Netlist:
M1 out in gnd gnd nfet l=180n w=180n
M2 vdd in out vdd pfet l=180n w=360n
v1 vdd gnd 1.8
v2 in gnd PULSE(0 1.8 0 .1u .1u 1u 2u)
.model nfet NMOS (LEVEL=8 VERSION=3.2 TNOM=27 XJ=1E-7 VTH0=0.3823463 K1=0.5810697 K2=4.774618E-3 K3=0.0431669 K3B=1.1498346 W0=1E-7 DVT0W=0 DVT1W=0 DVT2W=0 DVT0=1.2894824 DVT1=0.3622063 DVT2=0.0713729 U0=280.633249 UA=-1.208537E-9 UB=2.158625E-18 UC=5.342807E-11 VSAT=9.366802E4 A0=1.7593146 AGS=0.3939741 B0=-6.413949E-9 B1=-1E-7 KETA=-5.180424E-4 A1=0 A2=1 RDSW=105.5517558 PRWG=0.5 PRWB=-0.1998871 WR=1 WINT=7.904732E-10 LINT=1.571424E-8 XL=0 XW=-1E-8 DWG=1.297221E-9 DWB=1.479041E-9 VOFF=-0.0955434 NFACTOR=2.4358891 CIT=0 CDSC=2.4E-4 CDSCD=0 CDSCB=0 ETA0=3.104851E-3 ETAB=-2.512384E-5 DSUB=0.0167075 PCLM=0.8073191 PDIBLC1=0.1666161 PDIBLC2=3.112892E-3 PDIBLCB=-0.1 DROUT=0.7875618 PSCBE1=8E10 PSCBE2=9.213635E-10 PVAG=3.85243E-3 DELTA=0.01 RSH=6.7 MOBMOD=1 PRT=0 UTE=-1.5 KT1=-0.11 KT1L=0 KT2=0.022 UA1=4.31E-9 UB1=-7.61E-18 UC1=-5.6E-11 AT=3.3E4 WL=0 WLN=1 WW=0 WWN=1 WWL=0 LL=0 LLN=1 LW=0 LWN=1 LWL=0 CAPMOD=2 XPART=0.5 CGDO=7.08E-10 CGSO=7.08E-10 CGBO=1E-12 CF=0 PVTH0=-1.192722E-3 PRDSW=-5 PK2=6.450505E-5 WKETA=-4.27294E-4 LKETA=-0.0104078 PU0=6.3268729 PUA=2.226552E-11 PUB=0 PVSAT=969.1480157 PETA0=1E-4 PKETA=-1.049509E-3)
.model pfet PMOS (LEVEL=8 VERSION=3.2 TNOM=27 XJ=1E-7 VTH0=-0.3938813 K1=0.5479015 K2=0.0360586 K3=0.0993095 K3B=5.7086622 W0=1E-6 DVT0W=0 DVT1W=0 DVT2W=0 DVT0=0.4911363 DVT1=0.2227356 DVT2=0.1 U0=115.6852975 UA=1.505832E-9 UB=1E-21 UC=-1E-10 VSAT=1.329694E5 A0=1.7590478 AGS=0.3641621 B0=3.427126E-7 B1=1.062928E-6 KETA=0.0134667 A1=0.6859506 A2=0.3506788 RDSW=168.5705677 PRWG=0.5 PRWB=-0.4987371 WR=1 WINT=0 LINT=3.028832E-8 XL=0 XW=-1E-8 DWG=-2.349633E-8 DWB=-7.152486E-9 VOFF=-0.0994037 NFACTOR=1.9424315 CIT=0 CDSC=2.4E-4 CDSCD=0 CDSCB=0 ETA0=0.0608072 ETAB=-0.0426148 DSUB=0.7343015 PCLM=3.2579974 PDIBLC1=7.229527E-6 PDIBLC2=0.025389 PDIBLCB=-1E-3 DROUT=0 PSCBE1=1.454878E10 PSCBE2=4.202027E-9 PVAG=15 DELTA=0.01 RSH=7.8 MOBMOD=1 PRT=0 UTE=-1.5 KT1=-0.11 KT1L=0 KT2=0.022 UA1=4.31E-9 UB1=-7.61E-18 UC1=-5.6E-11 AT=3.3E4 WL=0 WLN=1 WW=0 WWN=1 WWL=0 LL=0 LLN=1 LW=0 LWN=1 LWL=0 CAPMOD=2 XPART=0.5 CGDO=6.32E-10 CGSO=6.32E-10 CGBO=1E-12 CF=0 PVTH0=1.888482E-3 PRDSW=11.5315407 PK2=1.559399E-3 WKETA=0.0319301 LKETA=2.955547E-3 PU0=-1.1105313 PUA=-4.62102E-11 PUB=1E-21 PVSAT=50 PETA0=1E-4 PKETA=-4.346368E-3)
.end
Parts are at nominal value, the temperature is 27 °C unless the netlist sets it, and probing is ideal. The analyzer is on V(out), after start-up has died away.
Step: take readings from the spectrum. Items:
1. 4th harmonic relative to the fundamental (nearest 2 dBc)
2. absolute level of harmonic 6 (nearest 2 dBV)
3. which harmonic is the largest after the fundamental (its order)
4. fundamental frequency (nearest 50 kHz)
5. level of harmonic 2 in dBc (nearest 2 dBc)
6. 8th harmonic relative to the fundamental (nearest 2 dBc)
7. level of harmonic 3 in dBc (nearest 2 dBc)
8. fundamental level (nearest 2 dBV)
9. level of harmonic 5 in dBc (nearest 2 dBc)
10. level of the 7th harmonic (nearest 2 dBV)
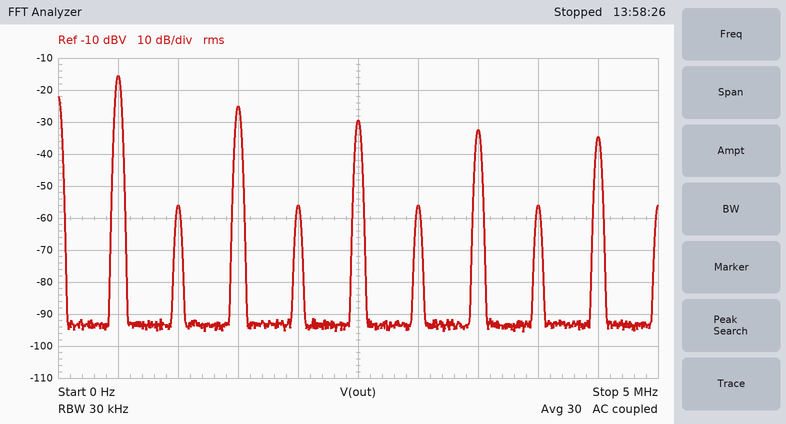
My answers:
-40 dBc
-56 dBV
3
500 kHz
-40 dBc
-40 dBc
-10 dBc
-16 dBV
-14 dBc
-32 dBV
